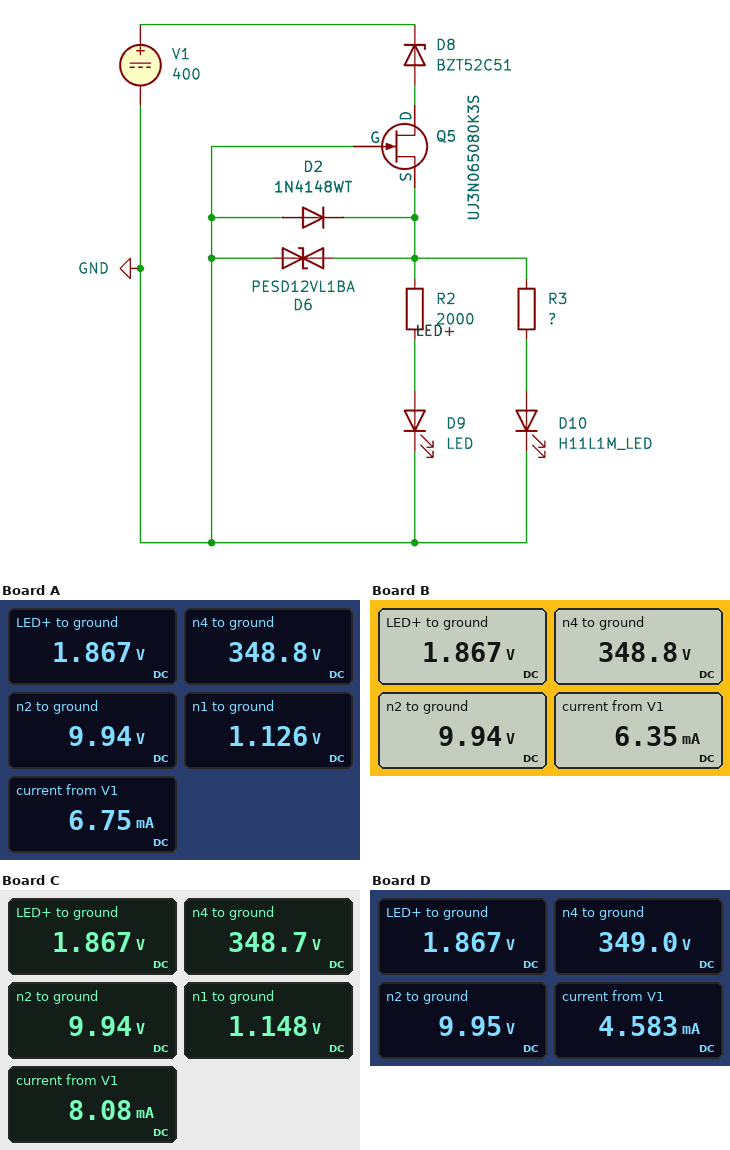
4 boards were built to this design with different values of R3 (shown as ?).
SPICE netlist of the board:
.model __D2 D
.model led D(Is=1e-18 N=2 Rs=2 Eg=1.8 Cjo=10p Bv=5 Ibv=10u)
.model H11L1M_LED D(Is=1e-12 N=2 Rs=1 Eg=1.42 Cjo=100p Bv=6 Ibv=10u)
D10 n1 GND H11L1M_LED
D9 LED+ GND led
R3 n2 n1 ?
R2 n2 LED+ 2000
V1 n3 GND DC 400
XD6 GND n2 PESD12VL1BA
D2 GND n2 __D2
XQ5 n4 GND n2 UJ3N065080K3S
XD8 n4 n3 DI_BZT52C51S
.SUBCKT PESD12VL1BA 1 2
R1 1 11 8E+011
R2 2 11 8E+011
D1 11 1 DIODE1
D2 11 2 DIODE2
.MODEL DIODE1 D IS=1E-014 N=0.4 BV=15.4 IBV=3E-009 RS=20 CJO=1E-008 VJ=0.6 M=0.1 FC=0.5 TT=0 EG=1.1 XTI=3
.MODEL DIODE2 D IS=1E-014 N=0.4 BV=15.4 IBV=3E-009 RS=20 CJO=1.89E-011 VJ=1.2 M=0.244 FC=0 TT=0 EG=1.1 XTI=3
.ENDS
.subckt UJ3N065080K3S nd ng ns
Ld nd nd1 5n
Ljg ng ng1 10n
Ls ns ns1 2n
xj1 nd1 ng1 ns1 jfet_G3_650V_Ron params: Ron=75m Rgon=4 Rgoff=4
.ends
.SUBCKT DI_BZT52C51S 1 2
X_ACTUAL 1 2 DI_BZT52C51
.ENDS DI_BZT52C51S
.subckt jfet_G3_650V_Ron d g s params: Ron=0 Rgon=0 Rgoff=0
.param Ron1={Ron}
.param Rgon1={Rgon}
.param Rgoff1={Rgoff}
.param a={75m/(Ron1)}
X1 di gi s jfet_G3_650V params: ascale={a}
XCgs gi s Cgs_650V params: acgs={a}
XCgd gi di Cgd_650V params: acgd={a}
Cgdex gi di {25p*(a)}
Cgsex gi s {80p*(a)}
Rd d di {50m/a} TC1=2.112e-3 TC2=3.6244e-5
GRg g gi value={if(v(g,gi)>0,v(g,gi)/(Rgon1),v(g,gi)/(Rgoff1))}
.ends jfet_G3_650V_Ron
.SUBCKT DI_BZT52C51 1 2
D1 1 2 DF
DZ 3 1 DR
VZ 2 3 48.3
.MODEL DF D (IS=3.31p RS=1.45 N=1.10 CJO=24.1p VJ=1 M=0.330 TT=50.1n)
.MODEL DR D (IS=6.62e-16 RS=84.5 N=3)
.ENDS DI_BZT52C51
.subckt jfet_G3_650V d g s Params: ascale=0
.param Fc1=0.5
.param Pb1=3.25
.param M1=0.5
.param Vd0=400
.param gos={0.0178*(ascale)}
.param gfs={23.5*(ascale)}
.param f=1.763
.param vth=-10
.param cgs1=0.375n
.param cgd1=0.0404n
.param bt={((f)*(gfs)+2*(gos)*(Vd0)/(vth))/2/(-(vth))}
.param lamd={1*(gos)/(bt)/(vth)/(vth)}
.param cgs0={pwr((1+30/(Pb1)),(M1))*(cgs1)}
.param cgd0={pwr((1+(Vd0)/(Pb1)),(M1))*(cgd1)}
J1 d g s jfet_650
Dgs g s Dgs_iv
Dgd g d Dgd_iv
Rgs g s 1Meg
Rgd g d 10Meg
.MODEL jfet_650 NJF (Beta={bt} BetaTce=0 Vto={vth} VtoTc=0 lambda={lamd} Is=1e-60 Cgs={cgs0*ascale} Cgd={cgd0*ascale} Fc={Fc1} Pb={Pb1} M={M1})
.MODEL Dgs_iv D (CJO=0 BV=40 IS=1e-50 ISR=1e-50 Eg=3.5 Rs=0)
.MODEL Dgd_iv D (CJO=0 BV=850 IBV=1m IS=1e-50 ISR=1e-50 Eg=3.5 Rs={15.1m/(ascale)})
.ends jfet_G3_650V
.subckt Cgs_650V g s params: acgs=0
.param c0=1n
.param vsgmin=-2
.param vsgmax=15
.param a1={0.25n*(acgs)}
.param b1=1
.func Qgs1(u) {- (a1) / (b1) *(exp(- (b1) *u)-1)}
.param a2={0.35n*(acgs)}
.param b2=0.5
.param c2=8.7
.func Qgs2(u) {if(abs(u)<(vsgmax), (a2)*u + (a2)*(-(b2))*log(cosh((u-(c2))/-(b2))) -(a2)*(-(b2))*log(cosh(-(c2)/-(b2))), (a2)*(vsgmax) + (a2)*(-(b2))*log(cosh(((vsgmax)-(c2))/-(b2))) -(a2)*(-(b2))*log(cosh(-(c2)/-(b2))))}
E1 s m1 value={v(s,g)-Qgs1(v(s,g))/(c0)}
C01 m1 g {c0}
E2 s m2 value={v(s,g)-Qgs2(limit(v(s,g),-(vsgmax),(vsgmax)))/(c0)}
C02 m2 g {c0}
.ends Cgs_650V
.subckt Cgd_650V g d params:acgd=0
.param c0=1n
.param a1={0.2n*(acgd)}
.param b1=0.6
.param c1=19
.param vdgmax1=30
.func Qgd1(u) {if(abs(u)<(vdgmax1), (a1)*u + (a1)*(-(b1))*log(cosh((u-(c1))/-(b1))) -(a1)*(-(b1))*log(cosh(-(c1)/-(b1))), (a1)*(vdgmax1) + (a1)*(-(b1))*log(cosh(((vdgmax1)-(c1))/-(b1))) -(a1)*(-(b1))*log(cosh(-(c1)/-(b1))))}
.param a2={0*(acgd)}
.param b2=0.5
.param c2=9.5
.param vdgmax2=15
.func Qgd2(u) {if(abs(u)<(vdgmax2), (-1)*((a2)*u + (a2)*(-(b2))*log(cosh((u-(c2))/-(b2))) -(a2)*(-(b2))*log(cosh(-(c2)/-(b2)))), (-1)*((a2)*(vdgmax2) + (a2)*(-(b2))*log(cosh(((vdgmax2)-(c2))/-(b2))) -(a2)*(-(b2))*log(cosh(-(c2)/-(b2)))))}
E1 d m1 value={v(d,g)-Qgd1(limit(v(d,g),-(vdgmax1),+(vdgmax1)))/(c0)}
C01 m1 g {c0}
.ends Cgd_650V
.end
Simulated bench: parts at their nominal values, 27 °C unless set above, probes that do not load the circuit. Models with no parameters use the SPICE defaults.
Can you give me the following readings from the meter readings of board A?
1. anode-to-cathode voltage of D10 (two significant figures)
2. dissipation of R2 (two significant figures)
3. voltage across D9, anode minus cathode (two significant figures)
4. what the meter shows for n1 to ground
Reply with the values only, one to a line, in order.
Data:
1.1 V
33 mW
1.9 V
1.126 V
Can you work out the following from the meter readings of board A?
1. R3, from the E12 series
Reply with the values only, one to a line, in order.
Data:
3.3 kΩ
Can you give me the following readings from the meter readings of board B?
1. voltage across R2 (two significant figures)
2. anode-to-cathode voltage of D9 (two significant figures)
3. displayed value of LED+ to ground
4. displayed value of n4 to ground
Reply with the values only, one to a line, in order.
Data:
8.1 V
1.9 V
1.867 V
348.8 V
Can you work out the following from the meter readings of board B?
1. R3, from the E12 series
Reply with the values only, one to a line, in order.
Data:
3.9 kΩ
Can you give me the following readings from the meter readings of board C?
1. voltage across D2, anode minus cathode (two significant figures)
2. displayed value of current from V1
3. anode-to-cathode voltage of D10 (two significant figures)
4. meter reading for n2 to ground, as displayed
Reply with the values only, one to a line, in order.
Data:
-9.9 V
8.08 mA
1.1 V
9.94 V
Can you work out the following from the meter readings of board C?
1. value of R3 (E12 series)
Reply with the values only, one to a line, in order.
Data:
2.2 kΩ
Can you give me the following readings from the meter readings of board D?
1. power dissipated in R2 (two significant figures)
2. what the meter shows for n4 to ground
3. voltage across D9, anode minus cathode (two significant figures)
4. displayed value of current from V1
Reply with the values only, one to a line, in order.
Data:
33 mW
349.0 V
1.9 V
4.583 mA
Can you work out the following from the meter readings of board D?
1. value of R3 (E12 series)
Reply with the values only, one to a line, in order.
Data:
18 kΩ
